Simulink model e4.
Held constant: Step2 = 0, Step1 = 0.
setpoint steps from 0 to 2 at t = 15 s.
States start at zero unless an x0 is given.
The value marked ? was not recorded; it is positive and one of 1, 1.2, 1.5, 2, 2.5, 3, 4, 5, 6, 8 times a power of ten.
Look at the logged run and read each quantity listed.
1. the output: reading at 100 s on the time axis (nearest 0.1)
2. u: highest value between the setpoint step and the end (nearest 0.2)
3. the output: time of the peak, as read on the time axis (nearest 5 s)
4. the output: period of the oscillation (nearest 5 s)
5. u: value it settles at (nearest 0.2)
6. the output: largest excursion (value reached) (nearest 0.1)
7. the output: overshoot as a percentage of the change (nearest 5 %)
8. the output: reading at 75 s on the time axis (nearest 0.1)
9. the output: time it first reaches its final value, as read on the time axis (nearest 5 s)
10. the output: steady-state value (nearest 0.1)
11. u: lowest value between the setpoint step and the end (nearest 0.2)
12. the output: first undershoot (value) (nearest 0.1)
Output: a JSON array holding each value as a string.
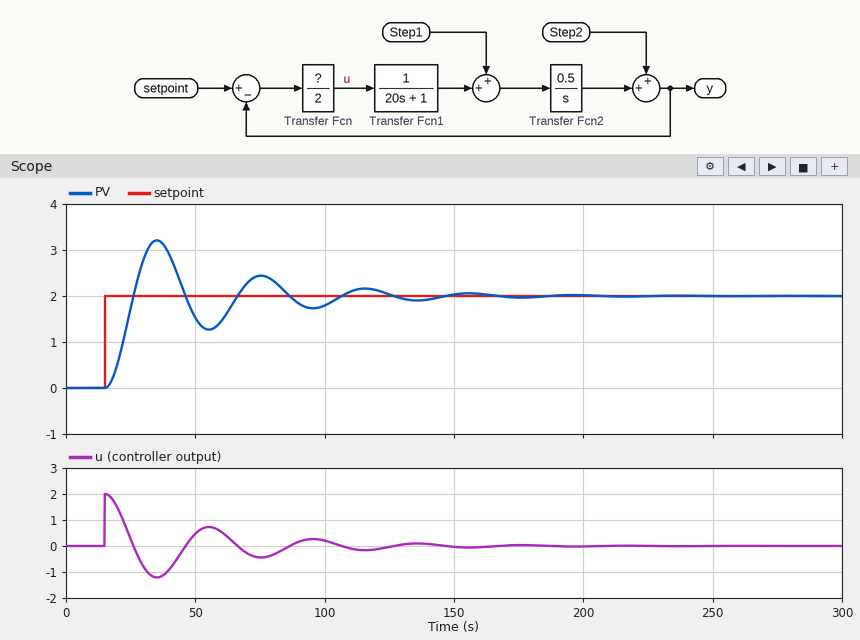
["1.8", "2.0", "35 s", "40 s", "0.0", "3.2", "60 %", "2.4", "25 s", "2.0", "-1.2", "1.3"]
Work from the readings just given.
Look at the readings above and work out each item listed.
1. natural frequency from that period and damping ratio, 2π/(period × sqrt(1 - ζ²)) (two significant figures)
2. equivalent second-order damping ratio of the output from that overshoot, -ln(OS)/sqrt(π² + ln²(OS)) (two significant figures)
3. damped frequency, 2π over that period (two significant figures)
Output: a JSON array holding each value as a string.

["0.16 rad/s", "0.16", "0.16 rad/s"]
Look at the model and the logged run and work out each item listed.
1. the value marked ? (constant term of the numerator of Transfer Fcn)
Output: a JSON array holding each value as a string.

["2"]
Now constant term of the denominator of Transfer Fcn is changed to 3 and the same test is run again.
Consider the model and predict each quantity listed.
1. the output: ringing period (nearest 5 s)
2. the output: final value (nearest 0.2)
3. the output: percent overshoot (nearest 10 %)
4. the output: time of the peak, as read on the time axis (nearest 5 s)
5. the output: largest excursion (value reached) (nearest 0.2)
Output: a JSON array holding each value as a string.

["50 s", "2.0", "50 %", "40 s", "3.0"]
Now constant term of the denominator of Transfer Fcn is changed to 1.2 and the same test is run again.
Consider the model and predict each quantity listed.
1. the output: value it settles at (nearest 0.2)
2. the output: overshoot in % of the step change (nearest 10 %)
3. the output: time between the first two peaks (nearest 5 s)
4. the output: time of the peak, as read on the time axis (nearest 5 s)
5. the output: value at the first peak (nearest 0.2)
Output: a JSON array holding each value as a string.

["2.0", "70 %", "30 s", "30 s", "3.4"]
